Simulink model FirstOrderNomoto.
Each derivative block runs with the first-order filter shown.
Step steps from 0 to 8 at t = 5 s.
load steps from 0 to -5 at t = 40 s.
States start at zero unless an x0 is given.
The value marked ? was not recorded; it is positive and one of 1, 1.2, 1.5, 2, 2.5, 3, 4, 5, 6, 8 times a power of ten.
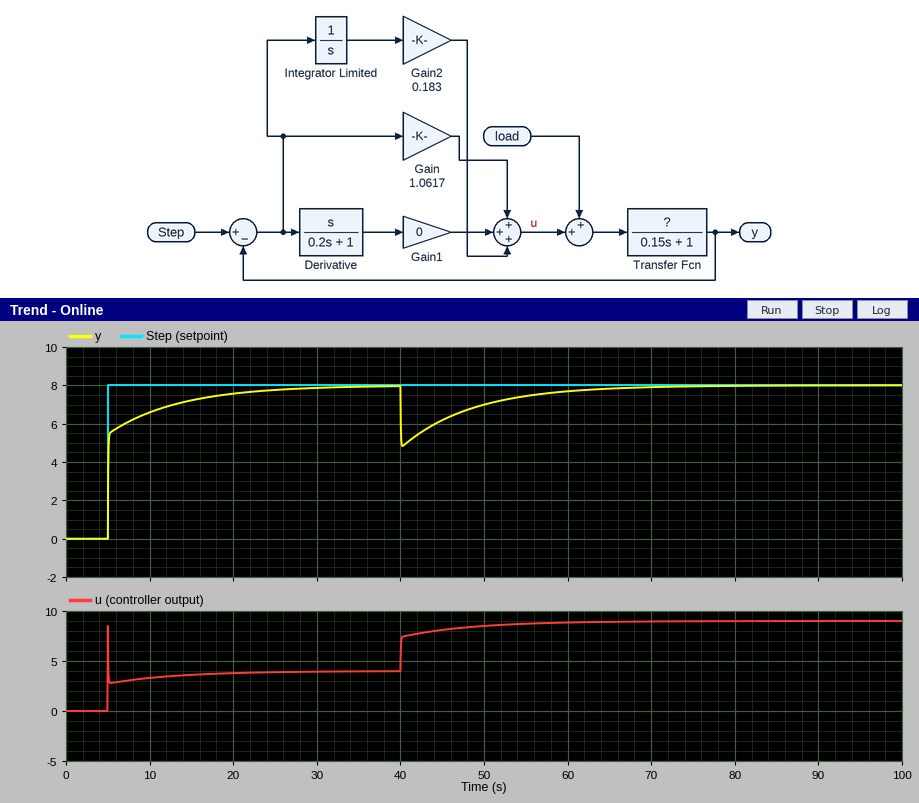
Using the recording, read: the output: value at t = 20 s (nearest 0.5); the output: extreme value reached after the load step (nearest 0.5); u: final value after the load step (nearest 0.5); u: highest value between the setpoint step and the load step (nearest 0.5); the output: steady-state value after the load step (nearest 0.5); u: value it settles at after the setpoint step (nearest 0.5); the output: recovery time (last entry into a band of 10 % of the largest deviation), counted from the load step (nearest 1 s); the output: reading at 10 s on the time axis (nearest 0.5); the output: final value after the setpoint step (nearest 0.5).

7.5
5.0
9.0
8.5
8.0
4.0
20 s
6.5
8.0
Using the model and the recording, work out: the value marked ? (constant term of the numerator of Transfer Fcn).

2
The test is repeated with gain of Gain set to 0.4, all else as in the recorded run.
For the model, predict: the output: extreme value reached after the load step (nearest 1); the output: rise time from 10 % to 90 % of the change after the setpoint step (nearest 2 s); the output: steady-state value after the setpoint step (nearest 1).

3
8 s
8
